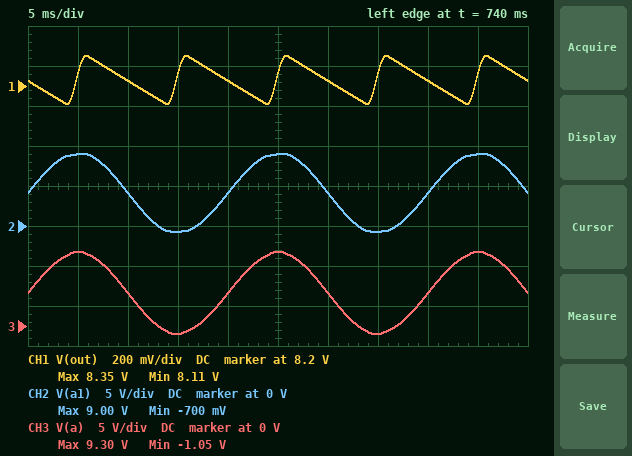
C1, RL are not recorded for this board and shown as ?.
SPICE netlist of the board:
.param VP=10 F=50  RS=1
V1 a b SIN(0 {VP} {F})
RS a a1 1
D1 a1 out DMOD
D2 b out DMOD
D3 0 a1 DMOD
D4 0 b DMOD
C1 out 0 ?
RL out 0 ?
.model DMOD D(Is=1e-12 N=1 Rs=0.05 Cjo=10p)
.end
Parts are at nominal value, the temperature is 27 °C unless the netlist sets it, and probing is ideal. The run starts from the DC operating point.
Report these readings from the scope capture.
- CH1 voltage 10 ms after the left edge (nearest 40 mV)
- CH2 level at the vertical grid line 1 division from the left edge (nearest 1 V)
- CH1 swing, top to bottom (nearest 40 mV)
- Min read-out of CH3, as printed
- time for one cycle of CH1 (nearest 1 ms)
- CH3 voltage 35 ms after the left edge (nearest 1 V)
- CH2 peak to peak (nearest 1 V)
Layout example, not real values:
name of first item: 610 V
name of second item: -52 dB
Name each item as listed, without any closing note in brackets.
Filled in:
CH1 voltage 10 ms after the left edge: 8.24 V
CH2 level at the vertical grid line 1 division from the left edge: 9 V
CH1 swing, top to bottom: 240 mV
Min read-out of CH3, as printed: -1.05 V
time for one cycle of CH1: 10 ms
CH3 voltage 35 ms after the left edge: -1 V
CH2 peak to peak: 10 V
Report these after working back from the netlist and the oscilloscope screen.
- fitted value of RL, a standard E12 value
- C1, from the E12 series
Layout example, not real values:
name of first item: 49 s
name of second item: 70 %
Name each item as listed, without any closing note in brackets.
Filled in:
fitted value of RL, a standard E12 value: 180 Ω
C1, from the E12 series: 1.5 mF
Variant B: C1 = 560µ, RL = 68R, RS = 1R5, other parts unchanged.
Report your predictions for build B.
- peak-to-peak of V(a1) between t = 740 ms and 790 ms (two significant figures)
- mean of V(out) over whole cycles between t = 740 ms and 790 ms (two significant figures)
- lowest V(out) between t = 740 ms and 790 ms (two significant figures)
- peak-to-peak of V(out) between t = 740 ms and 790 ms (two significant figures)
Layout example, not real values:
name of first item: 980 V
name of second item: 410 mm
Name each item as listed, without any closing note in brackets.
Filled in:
peak-to-peak of V(a1) between t = 740 ms and 790 ms: 9.6 V
mean of V(out) over whole cycles between t = 740 ms and 790 ms: 7.5 V
lowest V(out) between t = 740 ms and 790 ms: 6.8 V
peak-to-peak of V(out) between t = 740 ms and 790 ms: 1.4 V
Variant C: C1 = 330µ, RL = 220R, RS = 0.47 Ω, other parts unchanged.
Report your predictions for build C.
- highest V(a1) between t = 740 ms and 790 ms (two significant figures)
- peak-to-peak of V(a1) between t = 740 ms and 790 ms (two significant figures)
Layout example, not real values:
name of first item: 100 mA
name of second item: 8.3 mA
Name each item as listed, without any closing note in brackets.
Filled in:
highest V(a1) between t = 740 ms and 790 ms: 9.3 V
peak-to-peak of V(a1) between t = 740 ms and 790 ms: 10 V
